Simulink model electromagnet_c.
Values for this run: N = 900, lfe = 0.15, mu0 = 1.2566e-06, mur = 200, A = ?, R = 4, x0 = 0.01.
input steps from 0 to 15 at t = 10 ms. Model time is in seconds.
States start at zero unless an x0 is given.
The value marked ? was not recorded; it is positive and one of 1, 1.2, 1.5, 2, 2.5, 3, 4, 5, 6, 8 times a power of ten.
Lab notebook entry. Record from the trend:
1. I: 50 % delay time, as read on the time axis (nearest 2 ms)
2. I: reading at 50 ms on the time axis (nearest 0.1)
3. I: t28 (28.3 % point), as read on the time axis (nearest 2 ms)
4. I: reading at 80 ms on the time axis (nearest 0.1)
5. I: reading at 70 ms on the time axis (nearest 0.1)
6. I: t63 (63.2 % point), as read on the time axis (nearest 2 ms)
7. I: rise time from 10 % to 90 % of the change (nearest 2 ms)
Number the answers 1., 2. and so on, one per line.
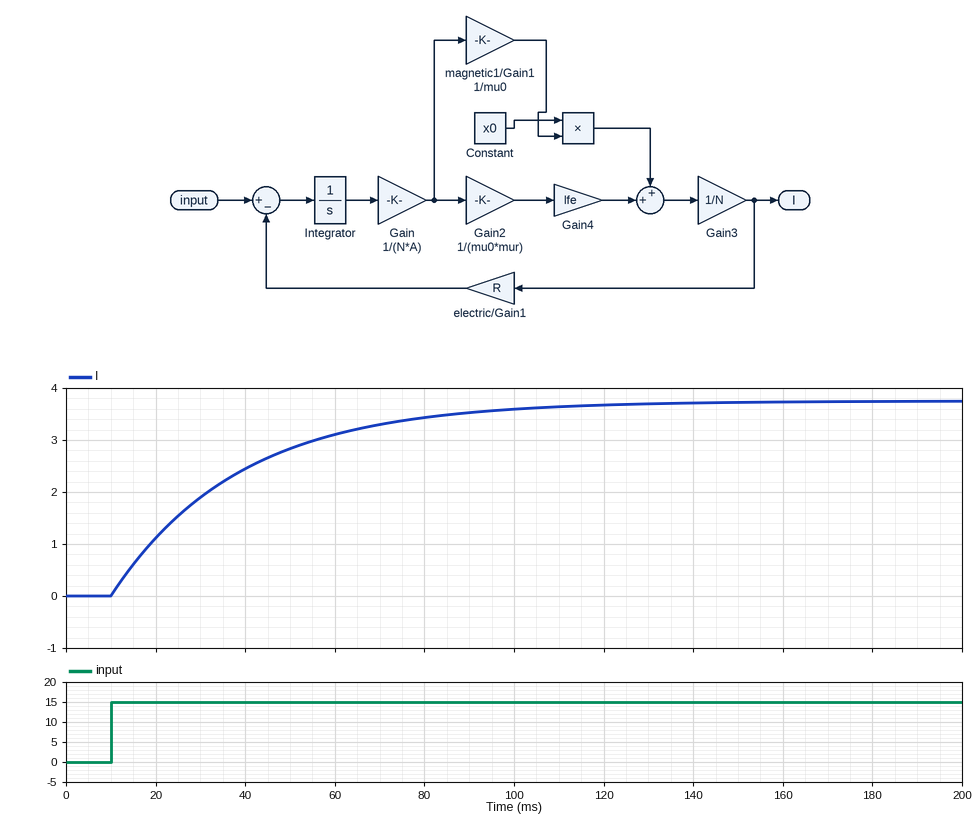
1. 30 ms
2. 2.8
3. 20 ms
4. 3.4
5. 3.3
6. 38 ms
7. 62 ms
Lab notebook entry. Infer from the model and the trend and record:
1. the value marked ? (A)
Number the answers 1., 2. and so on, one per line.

1. 0.0012
